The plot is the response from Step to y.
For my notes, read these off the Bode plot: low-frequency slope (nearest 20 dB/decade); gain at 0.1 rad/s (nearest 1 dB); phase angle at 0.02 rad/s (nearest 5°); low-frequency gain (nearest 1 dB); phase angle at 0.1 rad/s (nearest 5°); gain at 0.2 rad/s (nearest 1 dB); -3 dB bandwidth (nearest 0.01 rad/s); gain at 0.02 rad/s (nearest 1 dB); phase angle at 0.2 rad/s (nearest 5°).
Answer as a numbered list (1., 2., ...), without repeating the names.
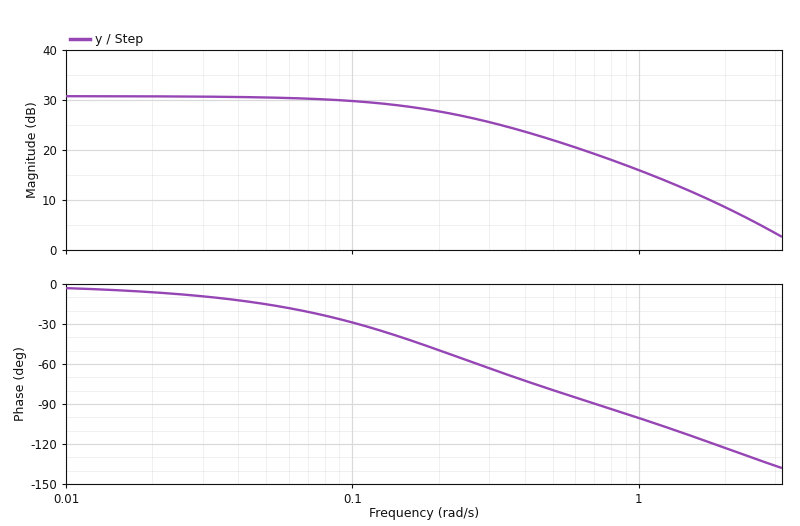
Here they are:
1. 0 dB/decade
2. 30 dB
3. -5°
4. 31 dB
5. -30°
6. 28 dB
7. 0.20 rad/s
8. 31 dB
9. -50°
